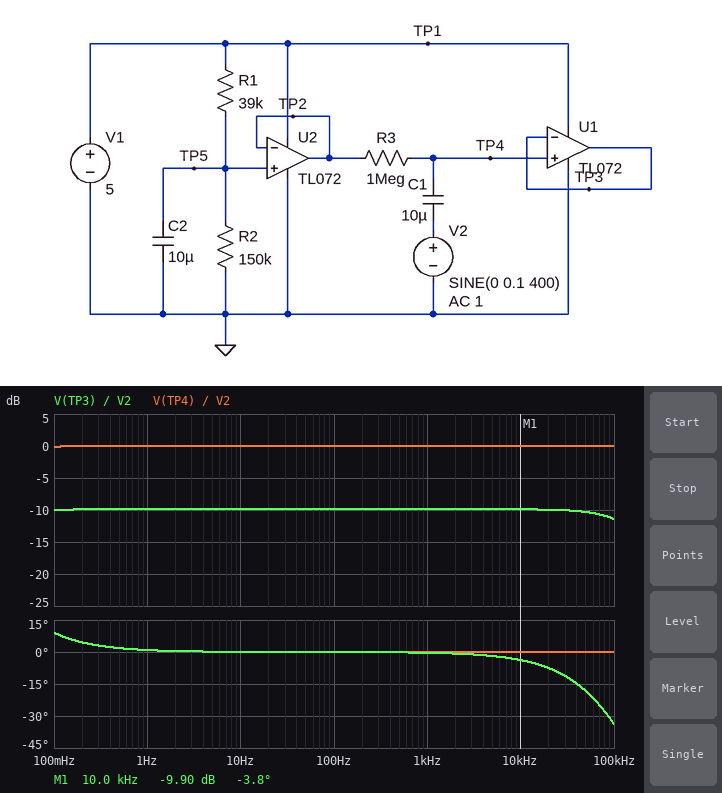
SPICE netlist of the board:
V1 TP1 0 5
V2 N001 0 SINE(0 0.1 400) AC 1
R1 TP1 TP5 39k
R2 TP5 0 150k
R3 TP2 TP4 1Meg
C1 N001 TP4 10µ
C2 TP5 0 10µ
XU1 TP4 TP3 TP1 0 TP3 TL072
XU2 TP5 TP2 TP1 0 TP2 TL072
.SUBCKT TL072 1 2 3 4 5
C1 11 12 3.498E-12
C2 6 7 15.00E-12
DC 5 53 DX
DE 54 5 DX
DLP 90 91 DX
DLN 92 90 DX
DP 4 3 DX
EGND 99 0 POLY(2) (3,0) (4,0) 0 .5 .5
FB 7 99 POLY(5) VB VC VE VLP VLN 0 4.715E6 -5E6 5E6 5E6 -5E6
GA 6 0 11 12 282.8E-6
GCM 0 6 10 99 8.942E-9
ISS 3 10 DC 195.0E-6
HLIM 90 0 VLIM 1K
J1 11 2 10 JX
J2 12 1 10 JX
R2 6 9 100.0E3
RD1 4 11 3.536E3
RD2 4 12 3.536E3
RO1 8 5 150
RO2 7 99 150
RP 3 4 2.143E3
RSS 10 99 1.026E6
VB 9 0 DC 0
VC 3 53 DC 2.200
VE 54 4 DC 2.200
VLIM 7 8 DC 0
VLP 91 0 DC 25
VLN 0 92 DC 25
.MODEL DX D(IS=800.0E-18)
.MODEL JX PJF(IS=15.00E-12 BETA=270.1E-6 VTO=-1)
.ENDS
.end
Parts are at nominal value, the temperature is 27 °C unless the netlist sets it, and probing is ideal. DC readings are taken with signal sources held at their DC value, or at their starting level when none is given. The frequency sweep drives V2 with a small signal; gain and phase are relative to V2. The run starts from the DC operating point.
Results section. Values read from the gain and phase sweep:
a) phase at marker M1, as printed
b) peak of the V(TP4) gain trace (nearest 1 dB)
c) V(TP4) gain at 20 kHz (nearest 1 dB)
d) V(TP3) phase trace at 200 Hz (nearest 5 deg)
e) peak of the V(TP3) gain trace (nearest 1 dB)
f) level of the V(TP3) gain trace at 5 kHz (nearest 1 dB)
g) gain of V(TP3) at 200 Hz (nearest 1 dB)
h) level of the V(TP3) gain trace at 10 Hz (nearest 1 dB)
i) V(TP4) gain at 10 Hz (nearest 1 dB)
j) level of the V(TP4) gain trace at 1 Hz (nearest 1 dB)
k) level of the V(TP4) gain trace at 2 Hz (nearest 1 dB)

-3.8 deg
0 dB
0 dB
0 deg
-10 dB
-10 dB
-10 dB
-10 dB
0 dB
0 dB
0 dB
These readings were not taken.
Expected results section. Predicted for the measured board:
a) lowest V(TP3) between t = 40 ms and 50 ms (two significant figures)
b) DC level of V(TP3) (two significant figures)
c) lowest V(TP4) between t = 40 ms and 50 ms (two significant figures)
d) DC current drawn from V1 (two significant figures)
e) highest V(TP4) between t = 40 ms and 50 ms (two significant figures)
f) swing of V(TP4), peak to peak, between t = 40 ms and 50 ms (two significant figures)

3.4 V
3.4 V
3.4 V
4.9 mA
3.6 V
200 mV
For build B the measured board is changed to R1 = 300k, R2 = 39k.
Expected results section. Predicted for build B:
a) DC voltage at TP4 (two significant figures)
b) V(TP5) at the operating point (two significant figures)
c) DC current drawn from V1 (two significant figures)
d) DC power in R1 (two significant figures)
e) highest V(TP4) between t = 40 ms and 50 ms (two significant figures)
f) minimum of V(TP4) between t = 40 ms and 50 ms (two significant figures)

1.5 V
590 mV
5.1 mA
65 µW
1.6 V
1.4 V
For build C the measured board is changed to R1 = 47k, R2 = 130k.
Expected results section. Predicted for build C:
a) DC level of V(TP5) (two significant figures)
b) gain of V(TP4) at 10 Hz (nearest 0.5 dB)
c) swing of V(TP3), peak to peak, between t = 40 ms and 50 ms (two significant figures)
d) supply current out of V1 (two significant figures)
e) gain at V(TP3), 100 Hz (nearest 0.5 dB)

3.7 V
0 dB
88 mV
5.0 mA
-8.5 dB
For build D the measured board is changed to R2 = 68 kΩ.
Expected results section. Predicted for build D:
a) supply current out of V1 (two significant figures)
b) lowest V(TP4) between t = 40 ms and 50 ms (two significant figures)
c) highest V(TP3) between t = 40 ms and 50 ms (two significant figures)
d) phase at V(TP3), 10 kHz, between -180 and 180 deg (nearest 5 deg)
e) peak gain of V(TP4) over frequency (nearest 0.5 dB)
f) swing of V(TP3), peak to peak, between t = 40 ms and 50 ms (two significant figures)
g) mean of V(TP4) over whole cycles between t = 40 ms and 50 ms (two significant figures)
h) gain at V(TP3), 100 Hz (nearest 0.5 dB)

5.1 mA
3.1 V
3.3 V
0 deg
0 dB
200 mV
3.2 V
0 dB
